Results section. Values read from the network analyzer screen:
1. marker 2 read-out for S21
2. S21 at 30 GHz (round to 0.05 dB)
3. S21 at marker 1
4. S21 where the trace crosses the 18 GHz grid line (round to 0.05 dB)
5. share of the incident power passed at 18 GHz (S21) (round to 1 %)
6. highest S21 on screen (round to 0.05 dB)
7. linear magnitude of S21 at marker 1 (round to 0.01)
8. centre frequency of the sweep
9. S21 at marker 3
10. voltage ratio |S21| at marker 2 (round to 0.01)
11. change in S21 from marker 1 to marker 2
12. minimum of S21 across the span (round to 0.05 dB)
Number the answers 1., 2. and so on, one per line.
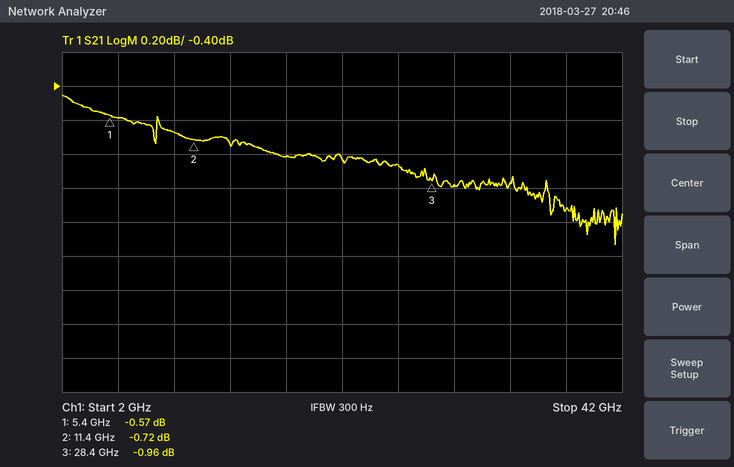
1. -0.72 dB
2. -1.00 dB
3. -0.57 dB
4. -0.80 dB
5. 83 %
6. -0.45 dB
7. 0.94
8. 22 GHz
9. -0.96 dB
10. 0.92
11. -0.15 dB
12. -1.35 dB
